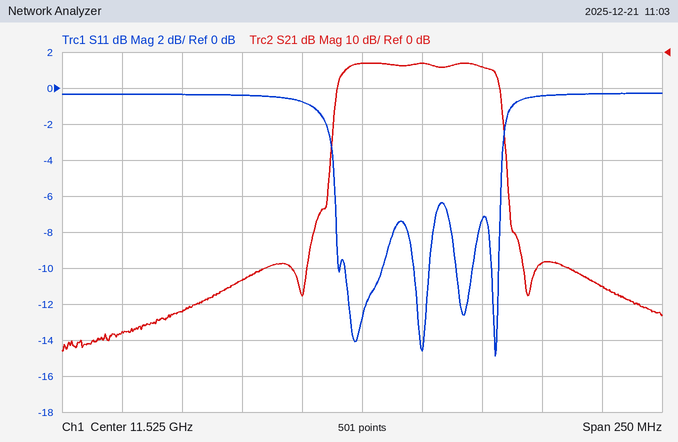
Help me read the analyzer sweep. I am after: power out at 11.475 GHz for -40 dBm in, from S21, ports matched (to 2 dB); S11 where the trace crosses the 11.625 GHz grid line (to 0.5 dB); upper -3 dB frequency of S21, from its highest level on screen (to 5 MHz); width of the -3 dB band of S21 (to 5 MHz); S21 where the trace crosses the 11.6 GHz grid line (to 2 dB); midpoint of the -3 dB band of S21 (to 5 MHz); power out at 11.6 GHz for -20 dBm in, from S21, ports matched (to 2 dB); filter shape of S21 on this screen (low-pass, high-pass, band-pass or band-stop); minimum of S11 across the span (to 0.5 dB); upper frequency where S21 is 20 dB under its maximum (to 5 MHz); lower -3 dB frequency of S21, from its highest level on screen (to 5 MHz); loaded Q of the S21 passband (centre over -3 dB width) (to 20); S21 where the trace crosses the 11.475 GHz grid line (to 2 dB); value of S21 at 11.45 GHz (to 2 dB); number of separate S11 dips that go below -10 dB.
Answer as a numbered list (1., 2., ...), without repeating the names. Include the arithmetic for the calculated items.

1. -40 dBm + (-64 dB) = -104 dBm
2. -0.5 dB
3. 11.580 GHz
4. 11.580 GHz − 11.515 GHz = 65 MHz
5. -58 dB
6. 11.550 GHz
7. -20 dBm + (-58 dB) = -78 dBm
8. band-pass
9. -15.0 dB
10. 11.585 GHz
11. 11.515 GHz
12. 11.5475 GHz / 65 MHz ≈ 178, so 180 to the nearest 20
13. -64 dB
14. -72 dB
15. 4
